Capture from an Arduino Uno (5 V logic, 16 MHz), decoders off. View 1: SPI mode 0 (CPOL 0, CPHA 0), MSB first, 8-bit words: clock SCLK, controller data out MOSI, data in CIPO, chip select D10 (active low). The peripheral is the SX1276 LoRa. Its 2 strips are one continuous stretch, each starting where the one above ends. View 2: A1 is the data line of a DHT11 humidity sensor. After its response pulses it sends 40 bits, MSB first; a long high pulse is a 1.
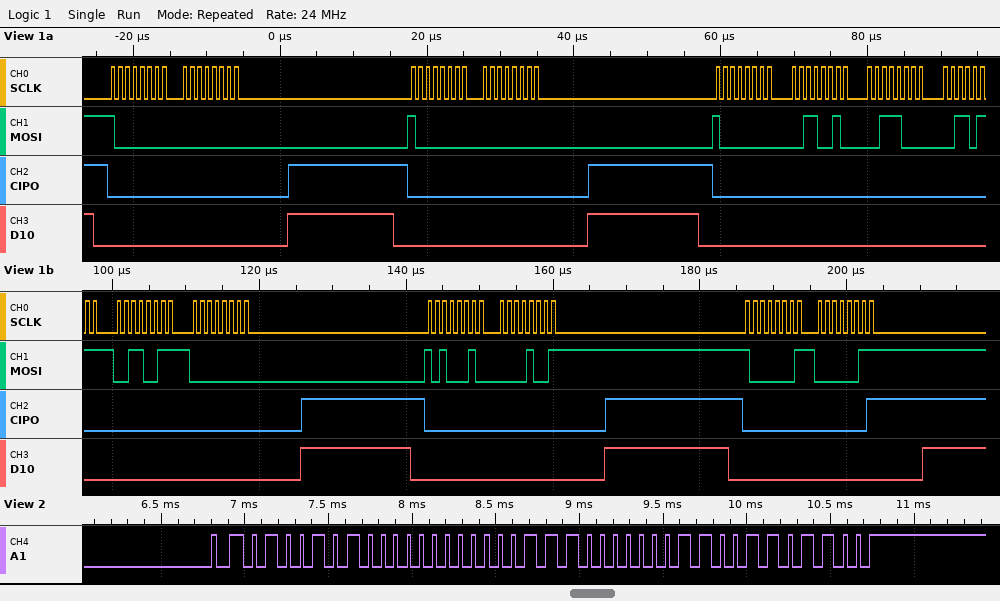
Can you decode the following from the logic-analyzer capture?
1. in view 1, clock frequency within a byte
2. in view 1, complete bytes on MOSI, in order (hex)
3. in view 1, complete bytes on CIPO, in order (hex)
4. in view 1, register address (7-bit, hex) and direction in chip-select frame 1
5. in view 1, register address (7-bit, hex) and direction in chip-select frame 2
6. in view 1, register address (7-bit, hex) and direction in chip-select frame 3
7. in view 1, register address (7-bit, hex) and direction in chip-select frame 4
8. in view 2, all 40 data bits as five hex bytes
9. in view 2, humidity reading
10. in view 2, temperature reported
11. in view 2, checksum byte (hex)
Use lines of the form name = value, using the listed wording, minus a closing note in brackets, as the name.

in view 1, clock frequency within a byte = 1 MHz
in view 1, complete bytes on MOSI, in order = 80 00 80 00 80 32 38 37 33 00 A2 09 81 03
in view 1, complete bytes on CIPO, in order = 00 00 00 00 00 00 00 00 00 00 00 00 00 01
in view 1, register address (7-bit, hex) and direction in chip-select frame 1 = 0x00 write
in view 1, register address (7-bit, hex) and direction in chip-select frame 2 = 0x00 write
in view 1, register address (7-bit, hex) and direction in chip-select frame 3 = 0x00 write
in view 1, register address (7-bit, hex) and direction in chip-select frame 4 = 0x22 write
in view 2, all 40 data bits as five hex bytes = 4A 00 1C 06 6C
in view 2, humidity reading = 74 %
in view 2, temperature reported = 28.6 °C
in view 2, checksum byte = 0x6C
